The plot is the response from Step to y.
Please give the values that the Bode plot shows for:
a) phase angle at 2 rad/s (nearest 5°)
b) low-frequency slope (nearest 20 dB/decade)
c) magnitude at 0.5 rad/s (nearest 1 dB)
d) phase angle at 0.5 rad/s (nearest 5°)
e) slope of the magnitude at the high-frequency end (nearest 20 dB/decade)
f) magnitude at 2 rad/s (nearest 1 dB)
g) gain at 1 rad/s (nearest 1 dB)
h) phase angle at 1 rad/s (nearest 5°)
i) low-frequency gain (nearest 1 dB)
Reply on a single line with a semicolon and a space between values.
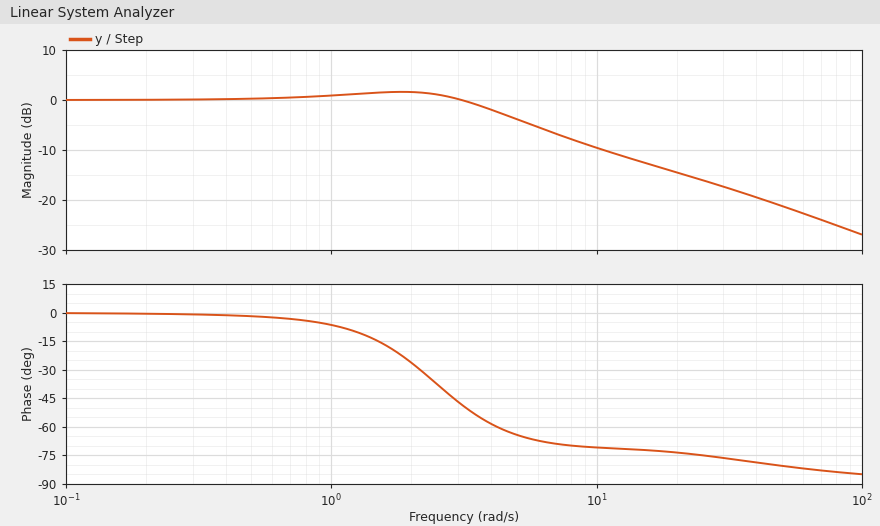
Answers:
-25°; 0 dB/decade; 0 dB; 0°; -20 dB/decade; 2 dB; 1 dB; -5°; 0 dB
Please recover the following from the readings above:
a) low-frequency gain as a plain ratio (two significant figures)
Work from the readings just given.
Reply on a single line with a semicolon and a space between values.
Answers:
1.0
